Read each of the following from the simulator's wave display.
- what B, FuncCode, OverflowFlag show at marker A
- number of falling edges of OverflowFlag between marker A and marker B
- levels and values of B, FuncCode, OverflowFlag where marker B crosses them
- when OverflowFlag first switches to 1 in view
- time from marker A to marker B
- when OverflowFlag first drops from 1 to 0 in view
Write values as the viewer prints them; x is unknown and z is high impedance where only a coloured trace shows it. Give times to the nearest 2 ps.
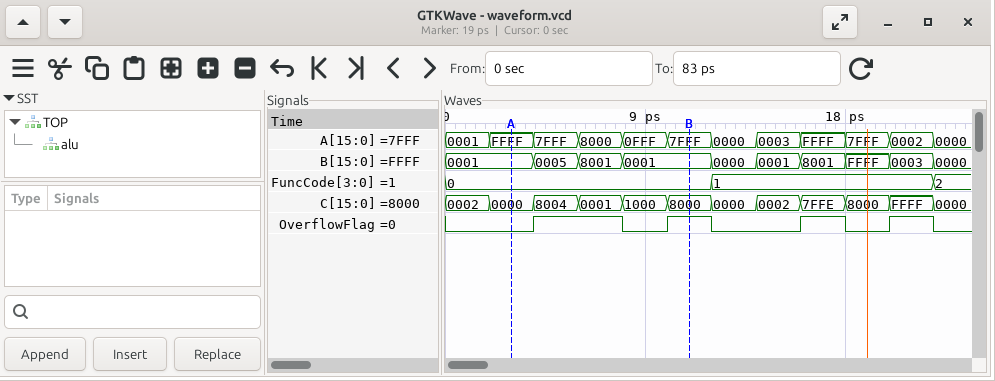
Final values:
B=0001, FuncCode=0, OverflowFlag=0
1
B=0001, FuncCode=0, OverflowFlag=1
4 ps
8 ps
8 ps
